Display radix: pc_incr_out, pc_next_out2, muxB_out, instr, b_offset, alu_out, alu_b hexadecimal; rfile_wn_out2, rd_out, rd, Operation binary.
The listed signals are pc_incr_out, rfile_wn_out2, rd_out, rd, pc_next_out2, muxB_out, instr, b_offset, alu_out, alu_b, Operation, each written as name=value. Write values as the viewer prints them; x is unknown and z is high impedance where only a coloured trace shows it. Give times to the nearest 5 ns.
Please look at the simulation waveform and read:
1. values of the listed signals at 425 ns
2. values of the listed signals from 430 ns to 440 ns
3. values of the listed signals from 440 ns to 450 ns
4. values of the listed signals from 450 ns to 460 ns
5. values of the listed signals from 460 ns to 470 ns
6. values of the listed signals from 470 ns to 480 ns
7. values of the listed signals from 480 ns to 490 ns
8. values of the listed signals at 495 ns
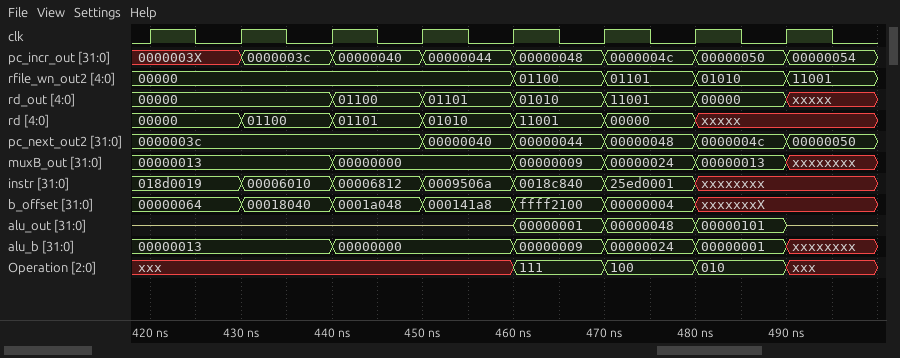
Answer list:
pc_incr_out=0000003X, rfile_wn_out2=00000, rd_out=00000, rd=00000, pc_next_out2=0000003c, muxB_out=00000013, instr=018d0019, b_offset=00000064, alu_out=z, alu_b=00000013, Operation=xxx
pc_incr_out=0000003c, rfile_wn_out2=00000, rd_out=00000, rd=01100, pc_next_out2=0000003c, muxB_out=00000013, instr=00006010, b_offset=00018040, alu_out=z, alu_b=00000013, Operation=xxx
pc_incr_out=00000040, rfile_wn_out2=00000, rd_out=01100, rd=01101, pc_next_out2=0000003c, muxB_out=00000000, instr=00006812, b_offset=0001a048, alu_out=z, alu_b=00000000, Operation=xxx
pc_incr_out=00000044, rfile_wn_out2=00000, rd_out=01101, rd=01010, pc_next_out2=00000040, muxB_out=00000000, instr=0009506a, b_offset=000141a8, alu_out=z, alu_b=00000000, Operation=xxx
pc_incr_out=00000048, rfile_wn_out2=01100, rd_out=01010, rd=11001, pc_next_out2=00000044, muxB_out=00000009, instr=0018c840, b_offset=ffff2100, alu_out=00000001, alu_b=00000009, Operation=111
pc_incr_out=0000004c, rfile_wn_out2=01101, rd_out=11001, rd=00000, pc_next_out2=00000048, muxB_out=00000024, instr=25ed0001, b_offset=00000004, alu_out=00000048, alu_b=00000024, Operation=100
pc_incr_out=00000050, rfile_wn_out2=01010, rd_out=00000, rd=xxxxx, pc_next_out2=0000004c, muxB_out=00000013, instr=xxxxxxxx, b_offset=xxxxxxxX, alu_out=00000101, alu_b=00000001, Operation=010
pc_incr_out=00000054, rfile_wn_out2=11001, rd_out=xxxxx, rd=xxxxx, pc_next_out2=00000050, muxB_out=xxxxxxxx, instr=xxxxxxxx, b_offset=xxxxxxxX, alu_out=z, alu_b=xxxxxxxx, Operation=xxx
